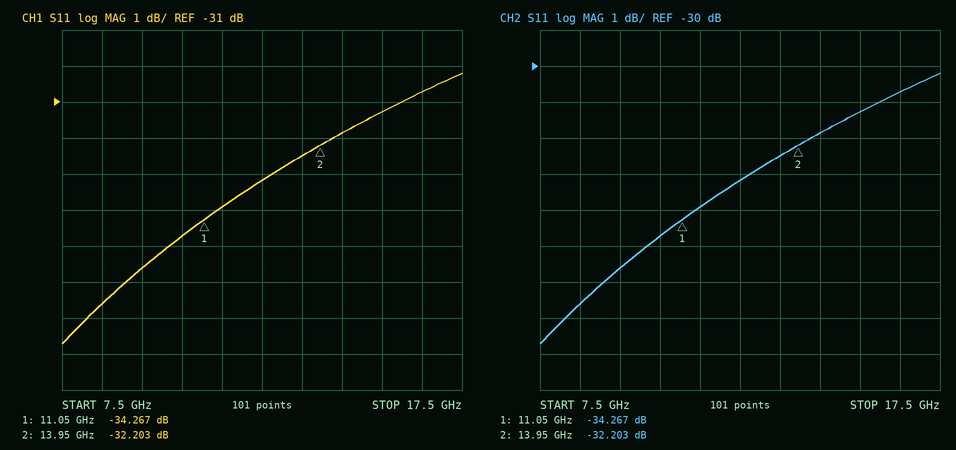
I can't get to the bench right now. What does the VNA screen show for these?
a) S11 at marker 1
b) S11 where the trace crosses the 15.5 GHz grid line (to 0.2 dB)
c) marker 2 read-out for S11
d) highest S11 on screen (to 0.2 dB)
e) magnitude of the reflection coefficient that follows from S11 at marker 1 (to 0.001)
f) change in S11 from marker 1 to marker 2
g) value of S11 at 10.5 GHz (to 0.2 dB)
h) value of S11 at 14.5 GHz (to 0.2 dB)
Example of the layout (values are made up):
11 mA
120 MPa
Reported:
-34.267 dB
-31.2 dB
-32.203 dB
-30.2 dB
0.019
2.064 dB
-34.8 dB
-31.8 dB
